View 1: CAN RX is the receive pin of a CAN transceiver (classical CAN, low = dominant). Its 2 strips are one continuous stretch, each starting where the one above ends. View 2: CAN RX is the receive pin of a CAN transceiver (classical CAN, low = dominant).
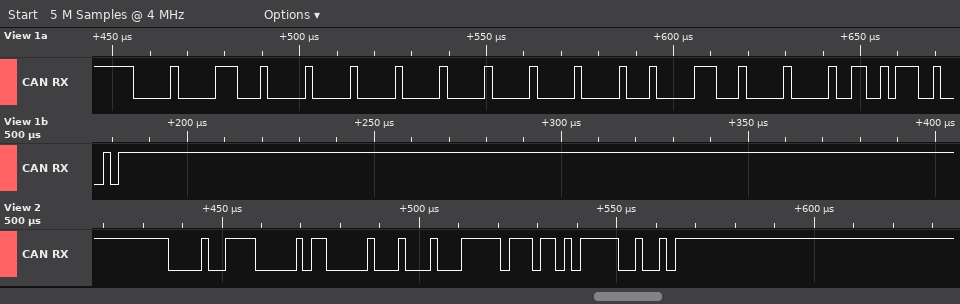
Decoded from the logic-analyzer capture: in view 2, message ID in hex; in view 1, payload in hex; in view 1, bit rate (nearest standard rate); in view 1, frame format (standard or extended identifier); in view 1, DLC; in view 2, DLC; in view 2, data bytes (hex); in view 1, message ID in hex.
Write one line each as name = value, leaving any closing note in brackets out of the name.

in view 2, message ID in hex = 0x09E
in view 1, payload in hex = 00 00 00 00 00 83 10 00
in view 1, bit rate = 500 kbit/s
in view 1, frame format = standard
in view 1, DLC = 8
in view 2, DLC = 3
in view 2, data bytes = 00 88 FF
in view 1, message ID in hex = 0x003
